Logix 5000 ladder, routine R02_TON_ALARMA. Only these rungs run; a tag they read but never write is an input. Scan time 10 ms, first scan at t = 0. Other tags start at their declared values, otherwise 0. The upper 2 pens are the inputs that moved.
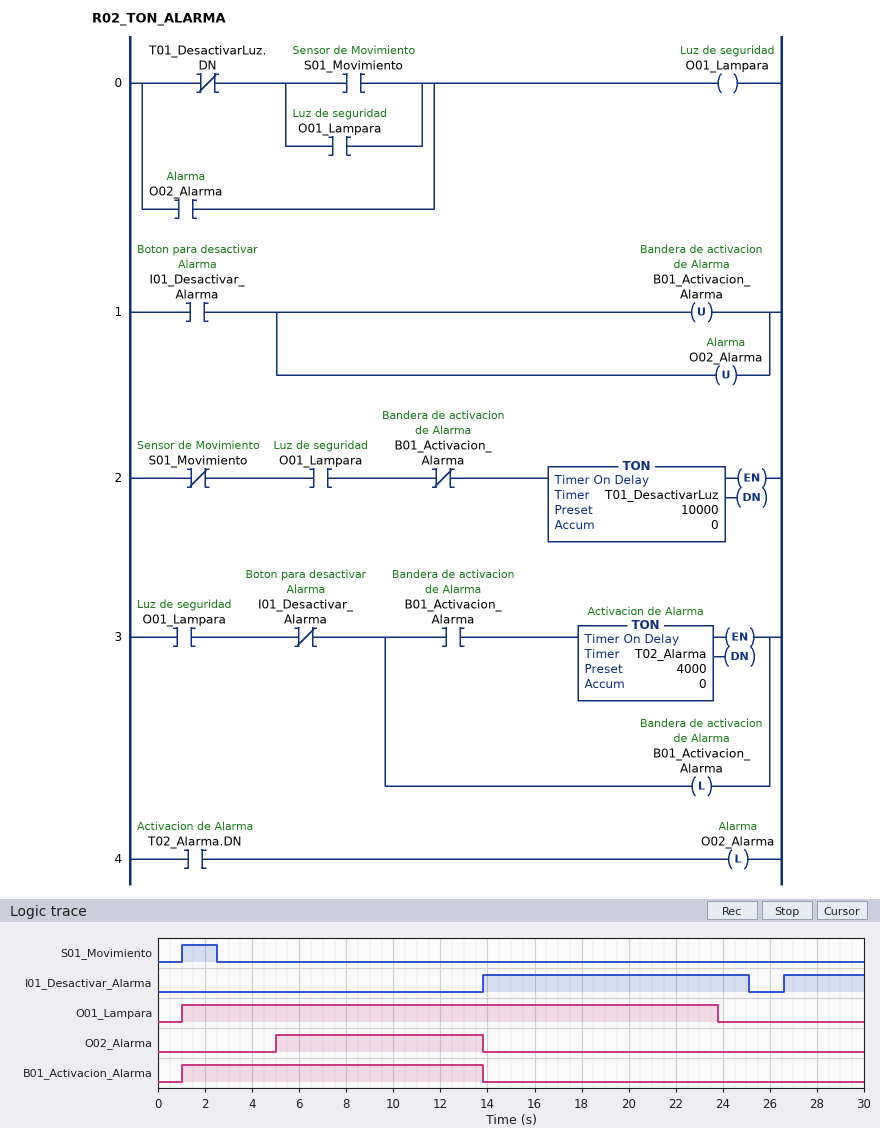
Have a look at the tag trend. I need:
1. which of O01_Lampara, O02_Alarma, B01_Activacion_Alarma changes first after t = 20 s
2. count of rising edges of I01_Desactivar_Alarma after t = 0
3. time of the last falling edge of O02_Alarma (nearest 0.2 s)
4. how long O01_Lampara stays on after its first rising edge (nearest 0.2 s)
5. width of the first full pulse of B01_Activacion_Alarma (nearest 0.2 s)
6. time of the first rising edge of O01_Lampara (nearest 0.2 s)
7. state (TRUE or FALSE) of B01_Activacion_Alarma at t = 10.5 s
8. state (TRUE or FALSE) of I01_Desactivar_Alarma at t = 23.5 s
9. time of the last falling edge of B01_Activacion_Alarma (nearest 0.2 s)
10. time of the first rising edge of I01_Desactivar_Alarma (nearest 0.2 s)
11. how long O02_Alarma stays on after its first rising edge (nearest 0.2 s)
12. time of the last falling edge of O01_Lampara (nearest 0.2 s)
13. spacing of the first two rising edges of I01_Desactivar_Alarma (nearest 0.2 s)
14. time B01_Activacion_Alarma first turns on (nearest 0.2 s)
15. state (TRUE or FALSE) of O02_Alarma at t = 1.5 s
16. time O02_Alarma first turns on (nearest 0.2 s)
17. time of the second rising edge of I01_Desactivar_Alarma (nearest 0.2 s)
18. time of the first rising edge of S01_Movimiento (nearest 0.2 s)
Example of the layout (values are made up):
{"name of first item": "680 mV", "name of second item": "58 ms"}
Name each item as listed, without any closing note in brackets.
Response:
{"which of O01_Lampara, O02_Alarma, B01_Activacion_Alarma changes first after t = 20 s": "O01_Lampara", "count of rising edges of I01_Desactivar_Alarma after t = 0": "2", "time of the last falling edge of O02_Alarma": "13.8 s", "how long O01_Lampara stays on after its first rising edge": "22.8 s", "width of the first full pulse of B01_Activacion_Alarma": "12.8 s", "time of the first rising edge of O01_Lampara": "1.0 s", "state (TRUE or FALSE) of B01_Activacion_Alarma at t = 10.5 s": "TRUE", "state (TRUE or FALSE) of I01_Desactivar_Alarma at t = 23.5 s": "TRUE", "time of the last falling edge of B01_Activacion_Alarma": "13.8 s", "time of the first rising edge of I01_Desactivar_Alarma": "13.8 s", "how long O02_Alarma stays on after its first rising edge": "8.8 s", "time of the last falling edge of O01_Lampara": "23.8 s", "spacing of the first two rising edges of I01_Desactivar_Alarma": "12.8 s", "time B01_Activacion_Alarma first turns on": "1.0 s", "state (TRUE or FALSE) of O02_Alarma at t = 1.5 s": "FALSE", "time O02_Alarma first turns on": "5.0 s", "time of the second rising edge of I01_Desactivar_Alarma": "26.6 s", "time of the first rising edge of S01_Movimiento": "1.0 s"}
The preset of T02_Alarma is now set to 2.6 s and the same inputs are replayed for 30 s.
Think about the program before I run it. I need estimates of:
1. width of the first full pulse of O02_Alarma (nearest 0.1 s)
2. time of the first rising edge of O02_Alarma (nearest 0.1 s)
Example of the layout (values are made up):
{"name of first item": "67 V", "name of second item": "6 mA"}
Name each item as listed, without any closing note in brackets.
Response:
{"width of the first full pulse of O02_Alarma": "10.2 s", "time of the first rising edge of O02_Alarma": "3.6 s"}
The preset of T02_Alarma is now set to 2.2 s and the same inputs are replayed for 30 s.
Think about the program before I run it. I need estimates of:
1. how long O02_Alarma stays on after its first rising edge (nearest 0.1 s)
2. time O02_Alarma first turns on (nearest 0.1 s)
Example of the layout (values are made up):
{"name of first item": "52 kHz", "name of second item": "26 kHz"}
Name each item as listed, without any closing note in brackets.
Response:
{"how long O02_Alarma stays on after its first rising edge": "10.6 s", "time O02_Alarma first turns on": "3.2 s"}
